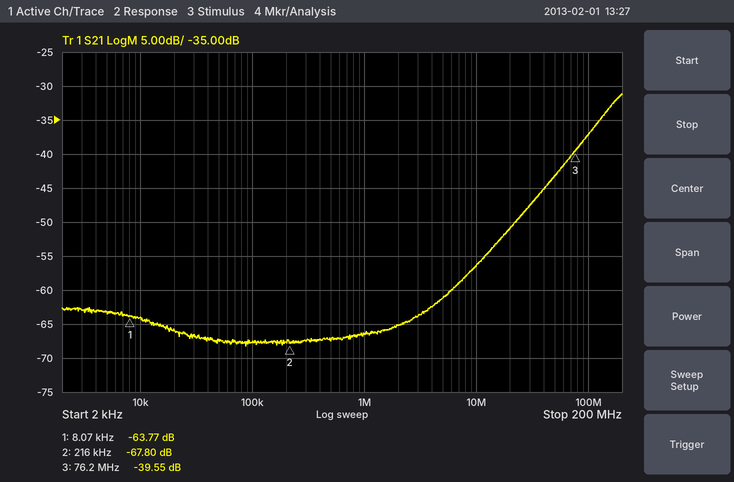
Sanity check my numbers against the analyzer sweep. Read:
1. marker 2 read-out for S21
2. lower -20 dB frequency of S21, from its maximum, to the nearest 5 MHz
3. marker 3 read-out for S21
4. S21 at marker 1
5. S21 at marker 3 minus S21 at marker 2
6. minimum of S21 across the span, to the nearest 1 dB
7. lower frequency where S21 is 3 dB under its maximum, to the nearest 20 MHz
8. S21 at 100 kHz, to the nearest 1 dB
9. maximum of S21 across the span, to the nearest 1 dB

-67.80 dB
20 MHz
-39.55 dB
-63.77 dB
28.25 dB
-68 dB
140 MHz
-68 dB
-31 dB
